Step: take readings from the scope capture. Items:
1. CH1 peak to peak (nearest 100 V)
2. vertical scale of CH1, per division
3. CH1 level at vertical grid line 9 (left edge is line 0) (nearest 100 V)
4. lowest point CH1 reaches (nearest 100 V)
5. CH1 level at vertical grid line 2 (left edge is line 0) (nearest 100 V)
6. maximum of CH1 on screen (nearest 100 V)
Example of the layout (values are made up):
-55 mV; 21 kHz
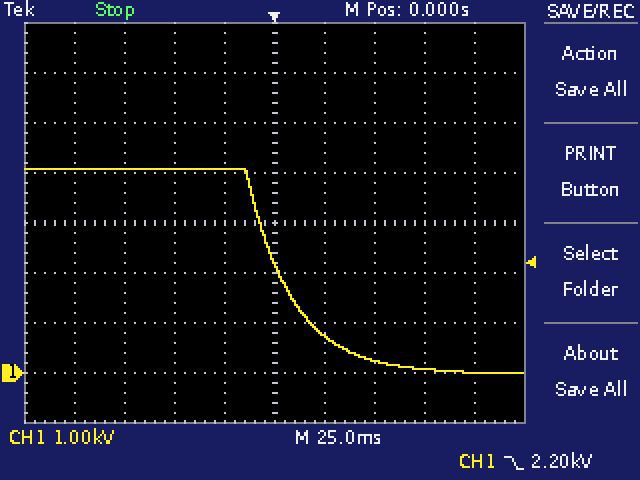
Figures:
4.1 kV; 1 kV; 0.0 kV; 0.0 kV; 4.1 kV; 4.1 kV
